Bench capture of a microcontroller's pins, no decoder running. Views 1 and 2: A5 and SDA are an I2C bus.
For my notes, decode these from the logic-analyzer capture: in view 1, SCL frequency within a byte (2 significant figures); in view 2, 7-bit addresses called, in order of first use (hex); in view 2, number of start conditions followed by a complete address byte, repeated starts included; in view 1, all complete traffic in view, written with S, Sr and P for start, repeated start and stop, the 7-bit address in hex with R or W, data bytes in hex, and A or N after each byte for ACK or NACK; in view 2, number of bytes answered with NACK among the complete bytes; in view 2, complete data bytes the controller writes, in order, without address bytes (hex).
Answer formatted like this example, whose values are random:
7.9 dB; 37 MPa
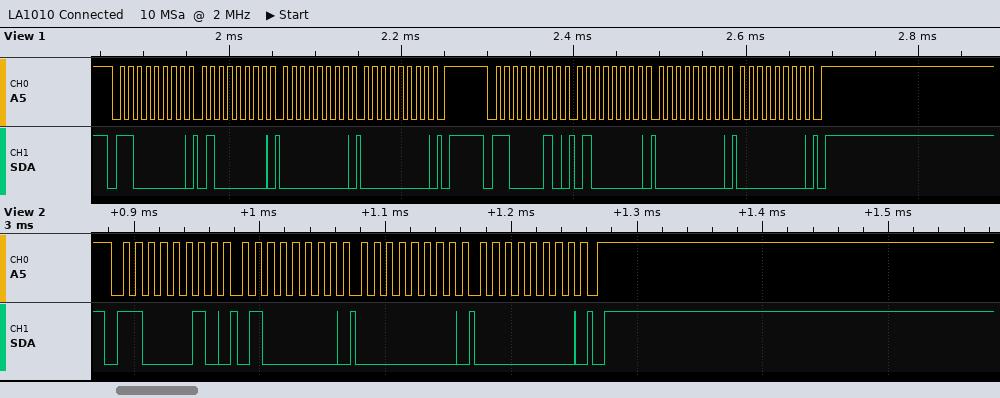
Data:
100 kHz; 0x61; 1; S 60W A 40 A 00 A 00 A P S 61W A 40 A 00 A 00 A P; 0; 40 00 00
